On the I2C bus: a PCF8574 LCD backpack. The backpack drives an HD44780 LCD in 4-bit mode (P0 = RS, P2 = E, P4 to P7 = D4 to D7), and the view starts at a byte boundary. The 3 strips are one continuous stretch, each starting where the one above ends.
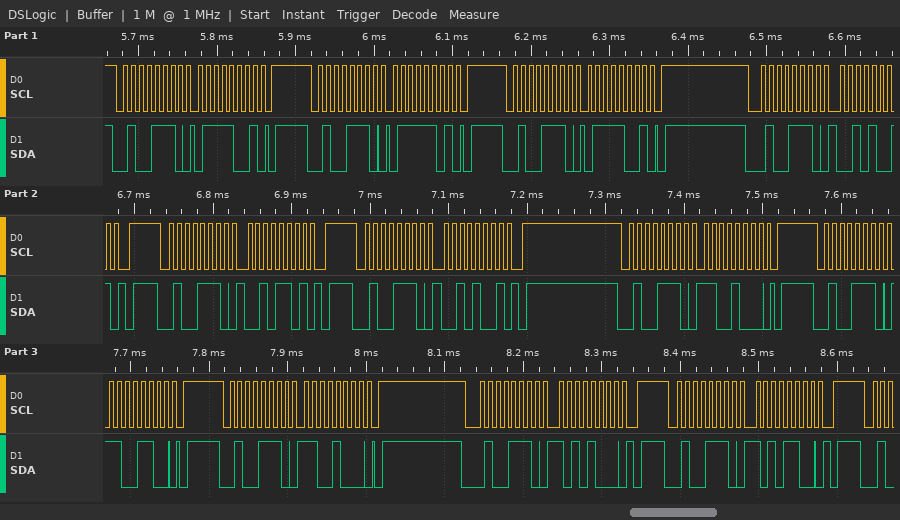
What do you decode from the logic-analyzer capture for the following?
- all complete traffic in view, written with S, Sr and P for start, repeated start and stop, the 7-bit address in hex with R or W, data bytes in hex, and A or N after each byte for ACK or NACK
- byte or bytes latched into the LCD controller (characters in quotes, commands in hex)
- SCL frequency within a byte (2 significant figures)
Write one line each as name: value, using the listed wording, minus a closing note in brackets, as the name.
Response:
all complete traffic in view, written with S, Sr and P for start, repeated start and stop, the 7-bit address in hex with R or W, data bytes in hex, and A or N after each byte for ACK or NACK: S 27W A 79 A P S 27W A 7D A P S 27W A 79 A P S 27W A 29 A P S 27W A 2D A P S 27W A 29 A P S 27W A C8 A P S 27W A CC A P S 27W A C8 A P S 27W A A8 A P S 27W A AC A P
byte or bytes latched into the LCD controller: 'r'
SCL frequency within a byte: 100 kHz
